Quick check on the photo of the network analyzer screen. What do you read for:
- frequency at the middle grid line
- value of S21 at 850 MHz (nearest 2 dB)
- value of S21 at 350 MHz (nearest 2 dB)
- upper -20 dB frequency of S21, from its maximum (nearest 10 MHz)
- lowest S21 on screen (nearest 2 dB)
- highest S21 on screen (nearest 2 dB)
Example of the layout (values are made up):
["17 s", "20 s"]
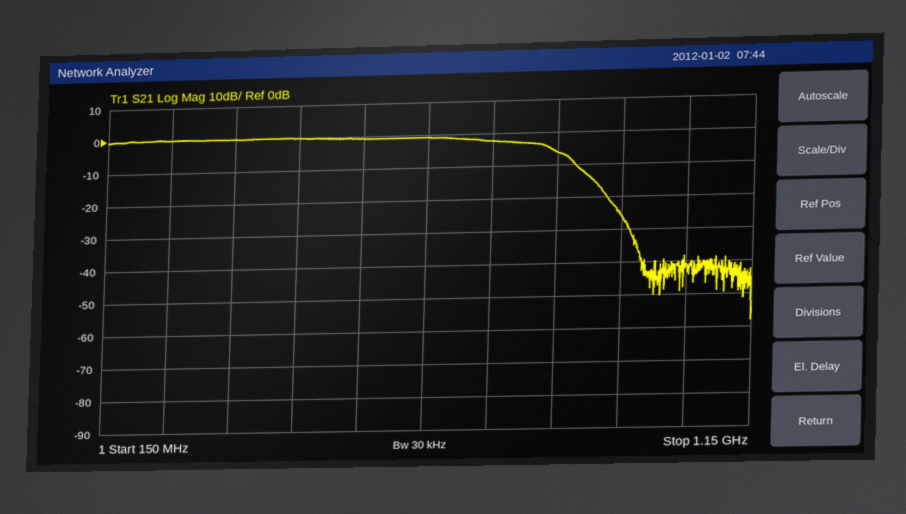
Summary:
["650 MHz", "-6 dB", "0 dB", "930 MHz", "-58 dB", "0 dB"]
